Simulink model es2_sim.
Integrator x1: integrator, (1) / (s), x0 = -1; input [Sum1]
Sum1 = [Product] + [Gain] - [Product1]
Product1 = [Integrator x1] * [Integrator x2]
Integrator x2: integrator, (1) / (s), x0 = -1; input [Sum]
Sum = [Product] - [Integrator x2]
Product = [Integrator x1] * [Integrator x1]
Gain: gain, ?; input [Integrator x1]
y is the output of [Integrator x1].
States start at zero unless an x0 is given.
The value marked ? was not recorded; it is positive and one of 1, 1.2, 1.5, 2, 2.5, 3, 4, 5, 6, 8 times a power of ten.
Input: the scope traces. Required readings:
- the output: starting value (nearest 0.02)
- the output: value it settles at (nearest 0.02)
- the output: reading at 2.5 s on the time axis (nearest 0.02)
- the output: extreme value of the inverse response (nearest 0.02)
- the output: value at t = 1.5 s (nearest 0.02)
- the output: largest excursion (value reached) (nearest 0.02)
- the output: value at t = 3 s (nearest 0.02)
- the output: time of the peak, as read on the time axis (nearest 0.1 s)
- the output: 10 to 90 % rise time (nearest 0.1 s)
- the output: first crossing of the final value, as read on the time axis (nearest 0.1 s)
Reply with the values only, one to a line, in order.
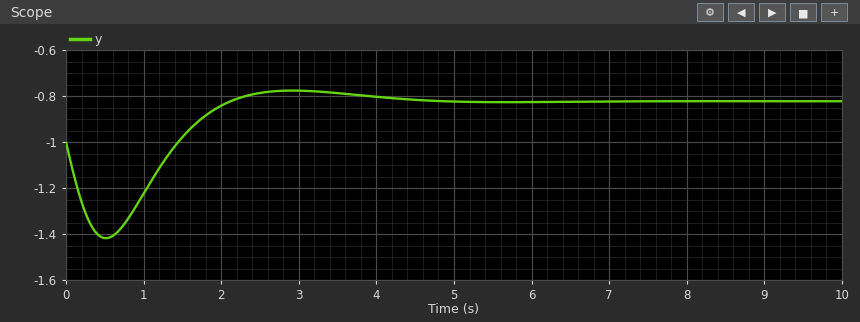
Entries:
-1.00
-0.82
-0.78
-1.42
-0.98
-0.78
-0.78
2.9 s
0.5 s
2.1 s
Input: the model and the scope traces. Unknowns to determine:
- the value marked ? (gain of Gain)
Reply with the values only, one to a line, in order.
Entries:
1.5
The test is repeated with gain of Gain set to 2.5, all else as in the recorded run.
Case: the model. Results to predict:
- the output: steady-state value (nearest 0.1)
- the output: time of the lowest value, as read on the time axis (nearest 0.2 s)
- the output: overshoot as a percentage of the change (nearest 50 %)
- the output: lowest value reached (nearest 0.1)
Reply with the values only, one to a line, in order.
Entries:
-1.2
0.6 s
500 %
-1.9
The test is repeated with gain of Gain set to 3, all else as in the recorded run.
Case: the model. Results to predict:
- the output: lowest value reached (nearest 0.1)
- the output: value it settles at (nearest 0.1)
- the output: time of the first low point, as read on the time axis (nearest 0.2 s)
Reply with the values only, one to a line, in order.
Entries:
-2.2
-1.3
0.6 s
